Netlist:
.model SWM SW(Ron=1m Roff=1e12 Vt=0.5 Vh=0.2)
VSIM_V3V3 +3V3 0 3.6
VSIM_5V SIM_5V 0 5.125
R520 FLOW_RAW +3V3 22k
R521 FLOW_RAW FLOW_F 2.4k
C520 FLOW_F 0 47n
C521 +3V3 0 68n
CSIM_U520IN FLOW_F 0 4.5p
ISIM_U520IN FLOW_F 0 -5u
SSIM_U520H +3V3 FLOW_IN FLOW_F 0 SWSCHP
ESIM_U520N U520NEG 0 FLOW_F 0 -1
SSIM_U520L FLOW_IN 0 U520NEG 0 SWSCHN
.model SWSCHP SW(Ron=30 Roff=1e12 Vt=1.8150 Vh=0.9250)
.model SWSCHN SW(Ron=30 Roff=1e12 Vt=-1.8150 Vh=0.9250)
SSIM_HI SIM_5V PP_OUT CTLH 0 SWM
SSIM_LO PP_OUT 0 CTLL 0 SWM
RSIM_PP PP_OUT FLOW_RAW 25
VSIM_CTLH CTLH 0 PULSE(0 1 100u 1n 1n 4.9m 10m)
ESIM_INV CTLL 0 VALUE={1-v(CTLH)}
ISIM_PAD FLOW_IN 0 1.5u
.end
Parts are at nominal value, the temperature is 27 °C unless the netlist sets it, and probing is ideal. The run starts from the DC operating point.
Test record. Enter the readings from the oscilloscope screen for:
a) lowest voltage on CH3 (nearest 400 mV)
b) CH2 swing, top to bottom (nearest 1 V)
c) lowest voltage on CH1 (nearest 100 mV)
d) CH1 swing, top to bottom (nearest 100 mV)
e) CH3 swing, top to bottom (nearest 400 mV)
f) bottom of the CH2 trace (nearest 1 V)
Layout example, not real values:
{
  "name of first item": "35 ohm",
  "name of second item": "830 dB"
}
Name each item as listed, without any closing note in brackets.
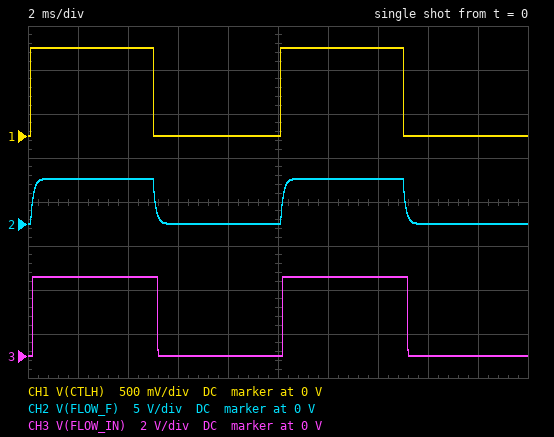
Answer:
{
  "lowest voltage on CH3": "0 V",
  "CH2 swing, top to bottom": "5 V",
  "lowest voltage on CH1": "0 V",
  "CH1 swing, top to bottom": "1.0 V",
  "CH3 swing, top to bottom": "3.6 V",
  "bottom of the CH2 trace": "0 V"
}
